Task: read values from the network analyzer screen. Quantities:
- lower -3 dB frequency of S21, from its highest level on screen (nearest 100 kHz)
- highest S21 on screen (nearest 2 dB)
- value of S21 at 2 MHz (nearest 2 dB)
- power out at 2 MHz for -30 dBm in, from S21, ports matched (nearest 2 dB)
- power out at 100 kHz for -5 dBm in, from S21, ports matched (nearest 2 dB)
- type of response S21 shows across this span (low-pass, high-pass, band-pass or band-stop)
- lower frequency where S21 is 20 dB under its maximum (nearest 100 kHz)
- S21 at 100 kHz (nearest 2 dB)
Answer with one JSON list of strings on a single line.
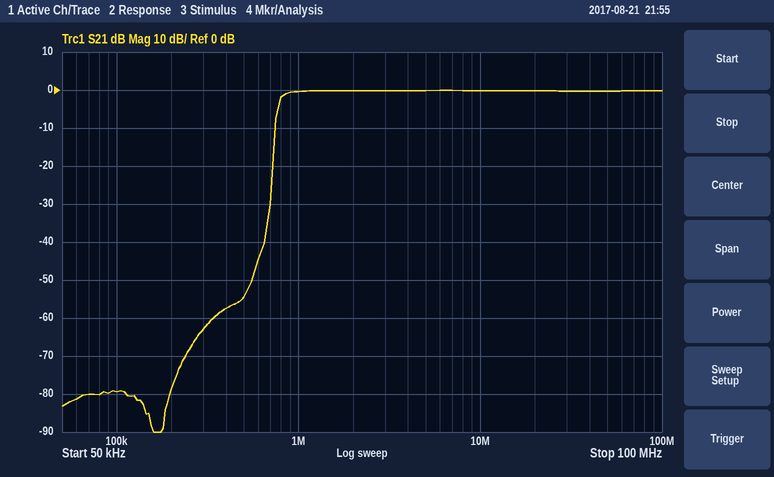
["800 kHz", "0 dB", "0 dB", "-30 dBm", "-84 dBm", "high-pass", "700 kHz", "-80 dB"]
